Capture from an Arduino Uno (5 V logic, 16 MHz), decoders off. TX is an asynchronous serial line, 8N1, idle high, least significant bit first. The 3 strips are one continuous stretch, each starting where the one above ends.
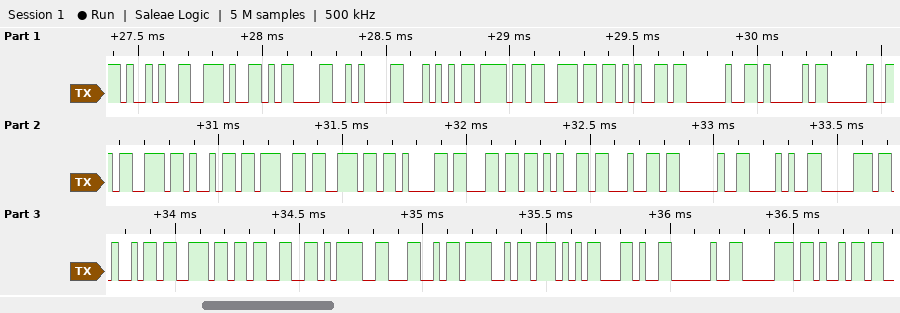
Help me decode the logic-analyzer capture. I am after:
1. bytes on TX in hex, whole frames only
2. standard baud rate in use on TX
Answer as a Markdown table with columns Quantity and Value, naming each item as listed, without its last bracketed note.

| Quantity | Value |
|---|---|
| bytes on TX in hex, whole frames only | 29 2E 0D 0A 54 6F 6E 65 20 41 20 73 69 67 6E 61 6C 65 64 20 28 70 69 6E 33 3D 4C 4F 57 2C 20 70 69 |
| standard baud rate in use on TX | 38400 baud |
